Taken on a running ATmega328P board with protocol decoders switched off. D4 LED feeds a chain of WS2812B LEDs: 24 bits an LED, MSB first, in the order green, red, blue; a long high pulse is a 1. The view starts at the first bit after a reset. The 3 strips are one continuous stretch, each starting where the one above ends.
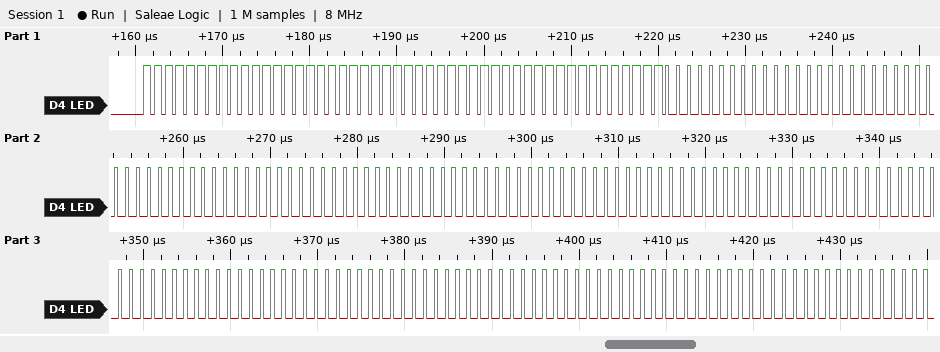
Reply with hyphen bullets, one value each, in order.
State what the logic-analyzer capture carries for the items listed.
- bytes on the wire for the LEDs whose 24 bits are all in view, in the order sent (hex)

- FF FF FF FF FF FF 00 00 00 00 00 00 00 00 00 00 00 00 00 00 00 00 00 00 00 00 00
